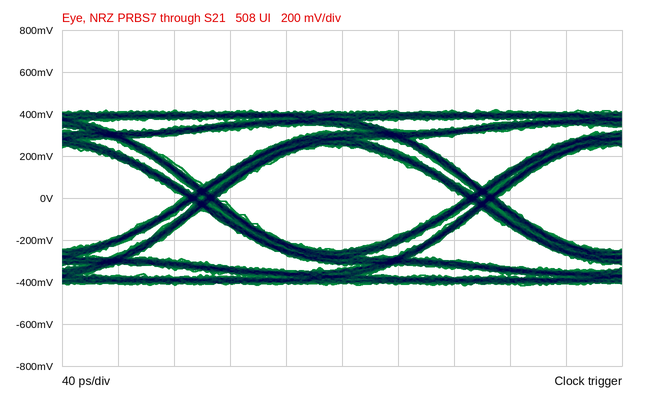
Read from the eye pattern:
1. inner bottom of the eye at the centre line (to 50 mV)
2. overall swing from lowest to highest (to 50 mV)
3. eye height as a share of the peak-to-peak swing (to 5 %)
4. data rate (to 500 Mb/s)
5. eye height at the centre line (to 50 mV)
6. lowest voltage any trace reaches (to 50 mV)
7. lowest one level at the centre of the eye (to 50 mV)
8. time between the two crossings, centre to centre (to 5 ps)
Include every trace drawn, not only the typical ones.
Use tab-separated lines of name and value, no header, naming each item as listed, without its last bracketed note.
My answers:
inner bottom of the eye at the centre line	-250 mV
overall swing from lowest to highest	850 mV
eye height as a share of the peak-to-peak swing	60 %
data rate	5.0 Gb/s
eye height at the centre line	500 mV
lowest voltage any trace reaches	-400 mV
lowest one level at the centre of the eye	250 mV
time between the two crossings, centre to centre	200 ps
